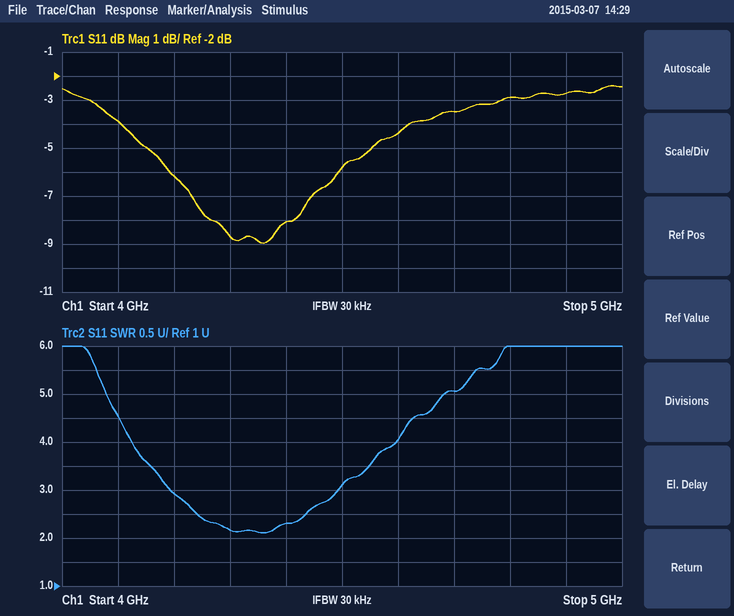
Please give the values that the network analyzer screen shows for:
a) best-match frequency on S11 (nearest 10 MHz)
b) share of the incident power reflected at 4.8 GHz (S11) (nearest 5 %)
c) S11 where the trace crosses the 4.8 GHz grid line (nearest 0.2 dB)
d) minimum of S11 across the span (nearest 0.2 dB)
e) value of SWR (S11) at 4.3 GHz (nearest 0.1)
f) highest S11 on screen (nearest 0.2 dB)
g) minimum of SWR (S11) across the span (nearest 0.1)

4.36 GHz
50 %
-2.8 dB
-9.0 dB
2.2
-2.4 dB
2.1
